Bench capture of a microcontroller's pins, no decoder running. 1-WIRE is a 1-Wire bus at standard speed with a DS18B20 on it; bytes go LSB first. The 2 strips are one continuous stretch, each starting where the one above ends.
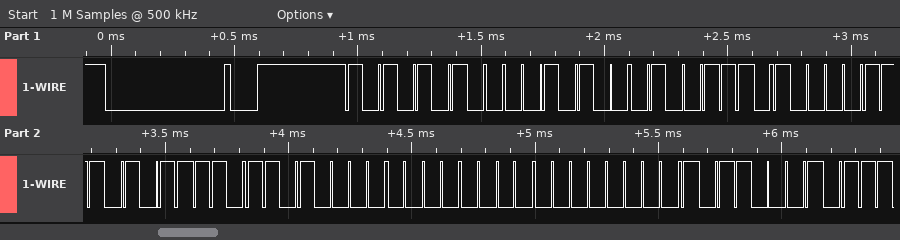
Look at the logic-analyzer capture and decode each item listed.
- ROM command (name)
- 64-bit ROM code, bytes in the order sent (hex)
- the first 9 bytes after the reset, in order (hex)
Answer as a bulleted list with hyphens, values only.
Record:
- Match ROM
- 28 72 E1 7A 0B 00 00 8D
- 55 28 72 E1 7A 0B 00 00 8D
